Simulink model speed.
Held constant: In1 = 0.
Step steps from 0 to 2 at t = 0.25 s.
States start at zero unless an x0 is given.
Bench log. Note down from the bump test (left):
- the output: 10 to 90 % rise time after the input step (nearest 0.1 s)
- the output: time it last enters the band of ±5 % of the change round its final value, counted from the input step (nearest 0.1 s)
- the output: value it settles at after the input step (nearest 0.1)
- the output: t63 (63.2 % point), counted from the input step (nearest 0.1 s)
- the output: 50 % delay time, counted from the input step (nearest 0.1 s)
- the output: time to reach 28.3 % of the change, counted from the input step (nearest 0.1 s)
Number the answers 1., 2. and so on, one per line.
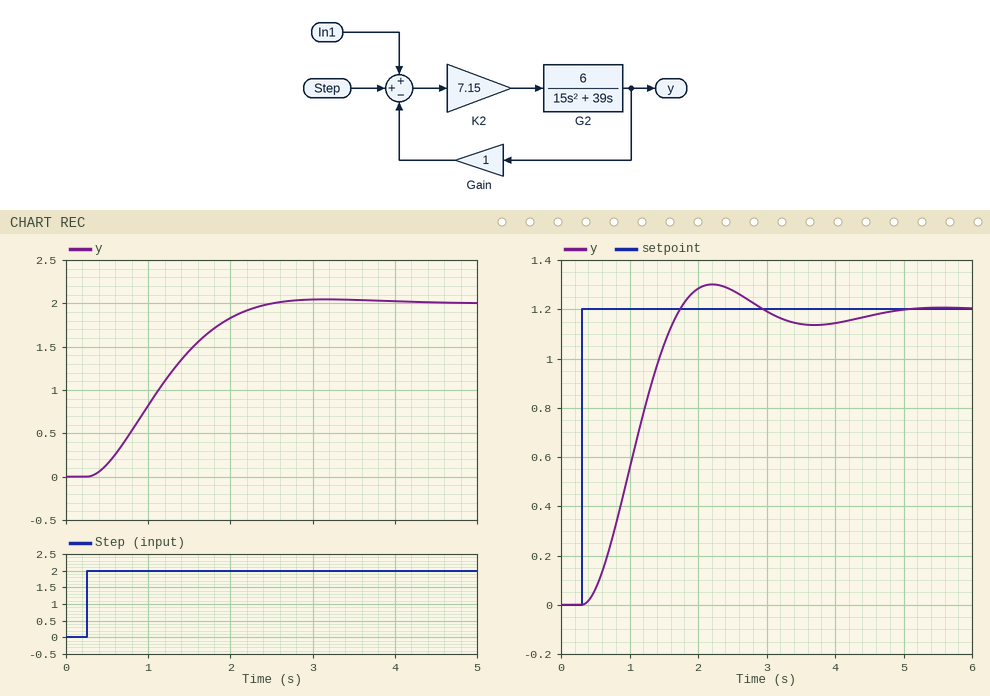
1. 1.4 s
2. 1.9 s
3. 2.0
4. 1.1 s
5. 0.9 s
6. 0.6 s
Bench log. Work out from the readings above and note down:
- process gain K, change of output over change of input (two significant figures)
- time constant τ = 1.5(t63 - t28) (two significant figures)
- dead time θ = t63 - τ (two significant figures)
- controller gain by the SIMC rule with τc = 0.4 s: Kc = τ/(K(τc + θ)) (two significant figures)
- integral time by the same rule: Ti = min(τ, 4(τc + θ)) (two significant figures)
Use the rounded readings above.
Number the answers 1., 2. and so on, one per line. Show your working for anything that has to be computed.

1. (2 - 0) / 2 = 1.0
2. 1.5 × (1.1 - 0.6) = 0.75 s
3. 1.1 - 0.75 = 0.35 s
4. 0.75 / (1 × (0.4 + 0.35)) = 1.0
5. min(0.75, 4 × (0.4 + 0.35)) = 0.75 s
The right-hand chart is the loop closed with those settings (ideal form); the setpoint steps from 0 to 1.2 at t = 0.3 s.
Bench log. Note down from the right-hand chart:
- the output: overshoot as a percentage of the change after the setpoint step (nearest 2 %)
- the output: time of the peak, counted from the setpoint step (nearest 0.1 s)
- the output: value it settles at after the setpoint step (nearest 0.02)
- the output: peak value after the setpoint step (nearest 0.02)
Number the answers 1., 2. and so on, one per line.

1. 8 %
2. 1.9 s
3. 1.20
4. 1.30
